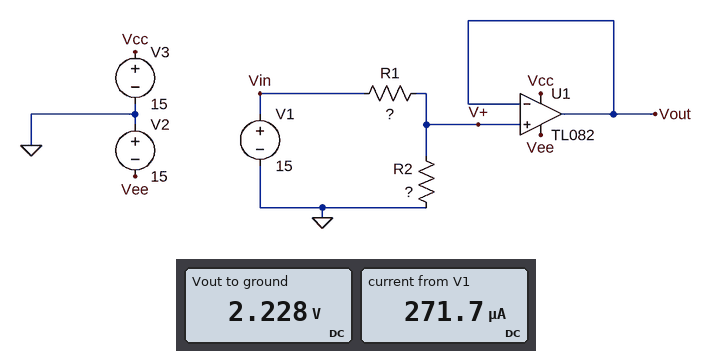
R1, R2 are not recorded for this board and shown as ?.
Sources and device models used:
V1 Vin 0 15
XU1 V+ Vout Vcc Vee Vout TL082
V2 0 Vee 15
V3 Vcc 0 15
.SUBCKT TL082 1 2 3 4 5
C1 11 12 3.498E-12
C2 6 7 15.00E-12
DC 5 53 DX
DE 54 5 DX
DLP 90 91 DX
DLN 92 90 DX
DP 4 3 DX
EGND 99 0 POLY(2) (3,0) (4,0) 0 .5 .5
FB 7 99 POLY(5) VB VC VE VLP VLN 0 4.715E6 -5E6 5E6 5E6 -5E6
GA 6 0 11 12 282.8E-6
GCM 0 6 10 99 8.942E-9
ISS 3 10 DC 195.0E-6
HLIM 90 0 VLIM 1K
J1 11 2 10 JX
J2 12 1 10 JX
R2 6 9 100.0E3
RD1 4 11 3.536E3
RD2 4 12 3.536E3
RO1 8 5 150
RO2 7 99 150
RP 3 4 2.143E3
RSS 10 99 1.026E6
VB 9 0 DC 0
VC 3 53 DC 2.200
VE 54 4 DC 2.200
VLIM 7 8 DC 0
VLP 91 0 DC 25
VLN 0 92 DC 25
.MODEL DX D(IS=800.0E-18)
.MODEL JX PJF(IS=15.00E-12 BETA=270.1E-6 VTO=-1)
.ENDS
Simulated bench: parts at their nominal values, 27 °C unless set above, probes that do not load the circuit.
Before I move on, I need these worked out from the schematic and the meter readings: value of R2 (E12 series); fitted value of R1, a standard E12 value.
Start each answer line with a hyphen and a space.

- 8.2 kΩ
- 47 kΩ
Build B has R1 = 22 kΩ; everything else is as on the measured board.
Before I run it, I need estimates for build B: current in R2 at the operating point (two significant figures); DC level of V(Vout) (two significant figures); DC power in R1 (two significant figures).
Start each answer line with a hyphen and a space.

- 500 µA
- 4.1 V
- 5.4 mW
